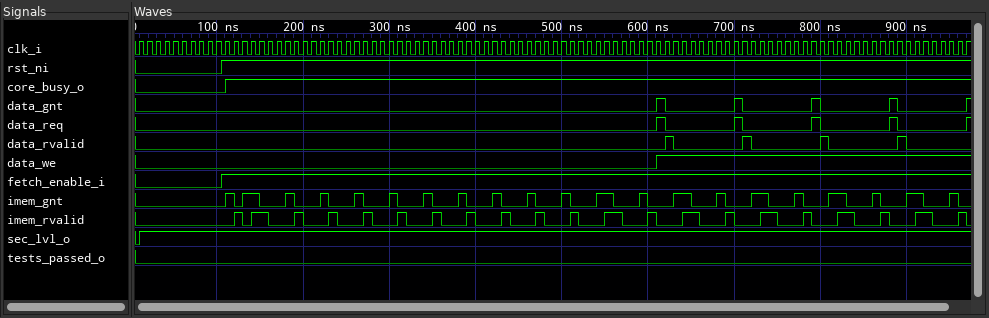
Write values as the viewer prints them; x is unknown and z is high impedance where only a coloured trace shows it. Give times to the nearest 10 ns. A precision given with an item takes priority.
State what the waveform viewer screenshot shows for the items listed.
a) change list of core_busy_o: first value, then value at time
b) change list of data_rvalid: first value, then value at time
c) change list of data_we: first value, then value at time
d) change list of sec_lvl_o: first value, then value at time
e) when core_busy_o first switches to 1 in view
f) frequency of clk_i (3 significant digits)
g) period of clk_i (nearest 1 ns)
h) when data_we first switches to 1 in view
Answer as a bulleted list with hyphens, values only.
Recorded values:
- 0, 1 at 110 ns
- 0, 1 at 620 ns, 0 at 630 ns, 1 at 710 ns, 0 at 720 ns, 1 at 800 ns, 0 at 810 ns, 1 at 890 ns, 0 at 900 ns
- 0, 1 at 610 ns
- 0, 1 at 10 ns
- 110 ns
- 100 MHz
- 10 ns
- 610 ns
